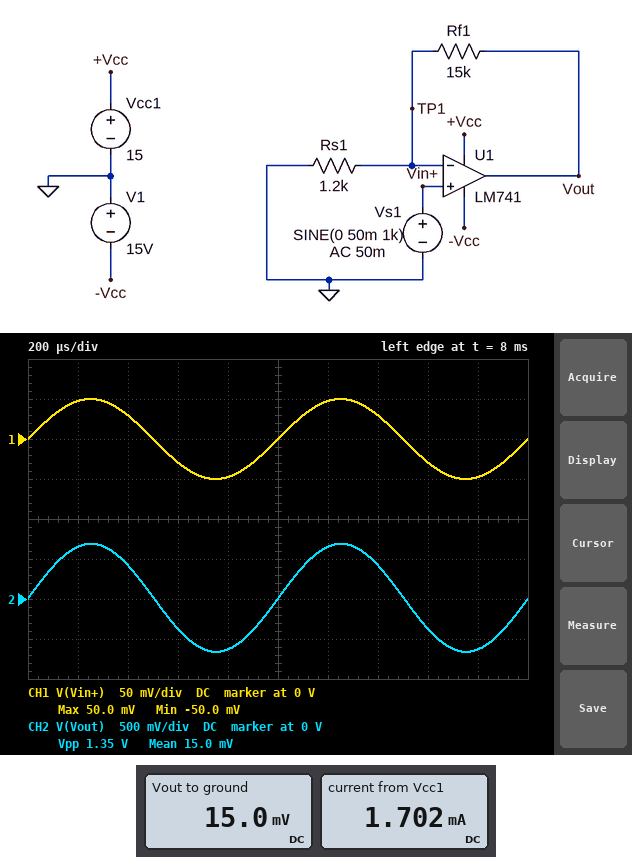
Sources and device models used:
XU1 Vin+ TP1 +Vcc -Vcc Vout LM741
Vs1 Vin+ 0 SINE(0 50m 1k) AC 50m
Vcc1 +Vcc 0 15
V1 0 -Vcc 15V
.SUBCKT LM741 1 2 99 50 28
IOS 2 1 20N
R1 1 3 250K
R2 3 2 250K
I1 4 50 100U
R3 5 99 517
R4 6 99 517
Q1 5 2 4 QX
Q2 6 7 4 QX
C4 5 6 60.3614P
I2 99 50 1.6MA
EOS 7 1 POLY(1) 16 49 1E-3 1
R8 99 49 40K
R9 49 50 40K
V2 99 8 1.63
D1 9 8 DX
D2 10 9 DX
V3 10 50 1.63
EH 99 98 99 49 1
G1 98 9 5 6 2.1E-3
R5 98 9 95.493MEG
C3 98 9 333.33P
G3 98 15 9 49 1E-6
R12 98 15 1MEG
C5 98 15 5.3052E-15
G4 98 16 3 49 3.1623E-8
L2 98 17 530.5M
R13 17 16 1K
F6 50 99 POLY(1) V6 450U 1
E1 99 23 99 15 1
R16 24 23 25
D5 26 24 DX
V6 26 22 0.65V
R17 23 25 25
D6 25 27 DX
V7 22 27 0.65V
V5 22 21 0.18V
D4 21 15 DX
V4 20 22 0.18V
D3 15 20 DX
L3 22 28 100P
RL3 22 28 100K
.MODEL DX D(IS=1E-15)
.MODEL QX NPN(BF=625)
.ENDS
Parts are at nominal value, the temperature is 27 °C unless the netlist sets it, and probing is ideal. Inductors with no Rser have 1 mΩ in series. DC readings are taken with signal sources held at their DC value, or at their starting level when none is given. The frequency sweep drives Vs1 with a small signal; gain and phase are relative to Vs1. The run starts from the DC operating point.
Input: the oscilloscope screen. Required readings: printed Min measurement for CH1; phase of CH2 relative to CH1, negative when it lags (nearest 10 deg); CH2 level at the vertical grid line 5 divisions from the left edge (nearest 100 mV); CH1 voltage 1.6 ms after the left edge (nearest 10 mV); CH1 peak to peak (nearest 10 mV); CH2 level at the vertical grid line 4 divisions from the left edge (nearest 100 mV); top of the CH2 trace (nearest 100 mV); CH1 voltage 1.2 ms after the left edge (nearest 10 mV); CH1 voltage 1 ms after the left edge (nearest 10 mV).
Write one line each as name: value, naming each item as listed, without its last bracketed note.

printed Min measurement for CH1: -50.0 mV
phase of CH2 relative to CH1, negative when it lags: 0 deg
CH2 level at the vertical grid line 5 divisions from the left edge: 0 V
CH1 voltage 1.6 ms after the left edge: -30 mV
CH1 peak to peak: 100 mV
CH2 level at the vertical grid line 4 divisions from the left edge: -600 mV
top of the CH2 trace: 700 mV
CH1 voltage 1.2 ms after the left edge: 50 mV
CH1 voltage 1 ms after the left edge: 0 V
